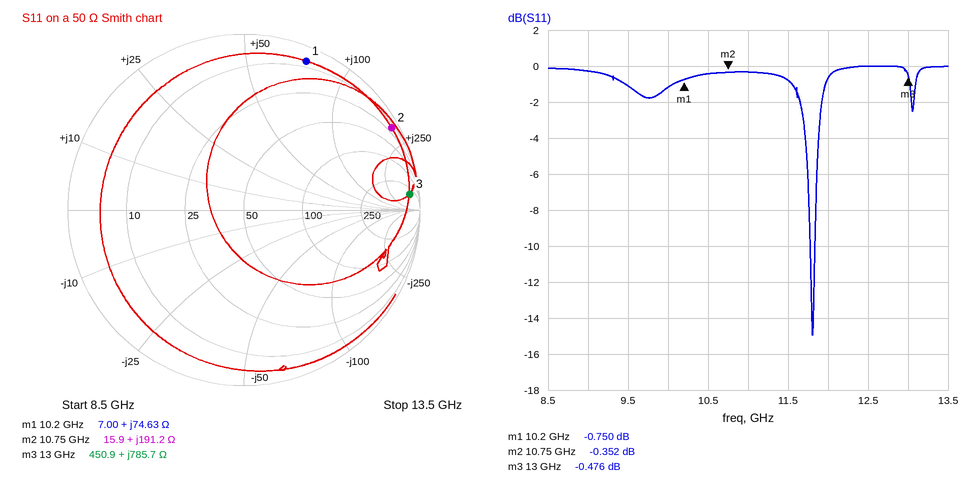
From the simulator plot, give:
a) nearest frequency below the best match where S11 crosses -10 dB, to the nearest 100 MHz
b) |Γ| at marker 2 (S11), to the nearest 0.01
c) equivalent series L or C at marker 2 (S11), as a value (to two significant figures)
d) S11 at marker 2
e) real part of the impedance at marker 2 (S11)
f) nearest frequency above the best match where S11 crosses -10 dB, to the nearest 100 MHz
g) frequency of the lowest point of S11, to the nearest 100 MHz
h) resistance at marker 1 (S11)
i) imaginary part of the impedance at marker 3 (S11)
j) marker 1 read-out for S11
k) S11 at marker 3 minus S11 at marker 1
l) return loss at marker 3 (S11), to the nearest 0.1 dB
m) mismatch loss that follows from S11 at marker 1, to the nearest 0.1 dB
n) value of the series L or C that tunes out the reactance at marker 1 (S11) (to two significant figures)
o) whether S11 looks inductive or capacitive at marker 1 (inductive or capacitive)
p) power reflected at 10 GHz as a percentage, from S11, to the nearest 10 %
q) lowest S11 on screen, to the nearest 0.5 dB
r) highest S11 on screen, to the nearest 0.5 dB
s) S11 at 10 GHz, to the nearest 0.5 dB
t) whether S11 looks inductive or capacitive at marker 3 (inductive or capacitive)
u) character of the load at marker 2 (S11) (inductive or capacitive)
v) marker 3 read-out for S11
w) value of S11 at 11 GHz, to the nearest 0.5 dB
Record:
11.8 GHz
0.96
2.8 nH
-0.352 dB
15.9 Ω
11.8 GHz
11.8 GHz
7.00 Ω
+785.7 Ω
-0.750 dB
0.274 dB
0.5 dB
8.0 dB
210 fF
inductive
80 %
-15.0 dB
0.0 dB
-1.0 dB
inductive
inductive
-0.476 dB
-0.5 dB
